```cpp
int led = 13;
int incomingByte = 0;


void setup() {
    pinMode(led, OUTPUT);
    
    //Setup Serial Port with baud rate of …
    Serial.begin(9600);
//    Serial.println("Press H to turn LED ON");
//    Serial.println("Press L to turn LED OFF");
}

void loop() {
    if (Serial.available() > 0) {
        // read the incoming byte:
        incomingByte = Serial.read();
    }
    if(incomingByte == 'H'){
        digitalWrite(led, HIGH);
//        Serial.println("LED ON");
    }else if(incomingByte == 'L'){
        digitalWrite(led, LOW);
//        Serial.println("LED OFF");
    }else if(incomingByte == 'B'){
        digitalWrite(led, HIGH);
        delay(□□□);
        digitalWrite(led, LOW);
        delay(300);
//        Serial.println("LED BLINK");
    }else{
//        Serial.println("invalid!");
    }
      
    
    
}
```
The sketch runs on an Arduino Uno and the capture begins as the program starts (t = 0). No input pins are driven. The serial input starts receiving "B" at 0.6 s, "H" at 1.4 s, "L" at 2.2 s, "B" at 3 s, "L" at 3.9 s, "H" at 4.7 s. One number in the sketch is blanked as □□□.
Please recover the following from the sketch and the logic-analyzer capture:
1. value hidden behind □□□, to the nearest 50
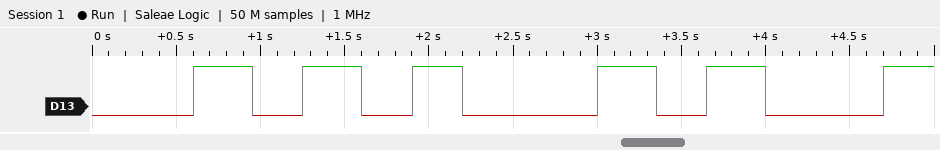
350
